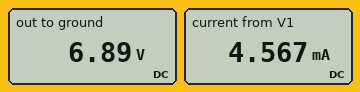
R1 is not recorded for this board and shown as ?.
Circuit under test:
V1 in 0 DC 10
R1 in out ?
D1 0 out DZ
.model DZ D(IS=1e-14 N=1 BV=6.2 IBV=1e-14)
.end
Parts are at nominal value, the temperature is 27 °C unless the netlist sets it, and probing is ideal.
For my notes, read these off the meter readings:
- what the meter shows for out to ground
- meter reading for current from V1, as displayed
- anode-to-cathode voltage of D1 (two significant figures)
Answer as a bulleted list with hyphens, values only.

- 6.89 V
- 4.567 mA
- -6.9 V
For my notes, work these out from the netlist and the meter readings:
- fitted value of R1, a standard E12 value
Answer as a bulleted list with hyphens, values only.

- 680 Ω
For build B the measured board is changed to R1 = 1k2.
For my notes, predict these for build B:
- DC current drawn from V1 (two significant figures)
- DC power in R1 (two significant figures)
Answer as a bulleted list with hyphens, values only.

- 2.6 mA
- 8.1 mW
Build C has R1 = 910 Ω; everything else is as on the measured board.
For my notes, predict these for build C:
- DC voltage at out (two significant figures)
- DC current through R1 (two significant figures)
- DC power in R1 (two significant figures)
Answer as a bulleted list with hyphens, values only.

- 6.9 V
- 3.4 mA
- 11 mW
